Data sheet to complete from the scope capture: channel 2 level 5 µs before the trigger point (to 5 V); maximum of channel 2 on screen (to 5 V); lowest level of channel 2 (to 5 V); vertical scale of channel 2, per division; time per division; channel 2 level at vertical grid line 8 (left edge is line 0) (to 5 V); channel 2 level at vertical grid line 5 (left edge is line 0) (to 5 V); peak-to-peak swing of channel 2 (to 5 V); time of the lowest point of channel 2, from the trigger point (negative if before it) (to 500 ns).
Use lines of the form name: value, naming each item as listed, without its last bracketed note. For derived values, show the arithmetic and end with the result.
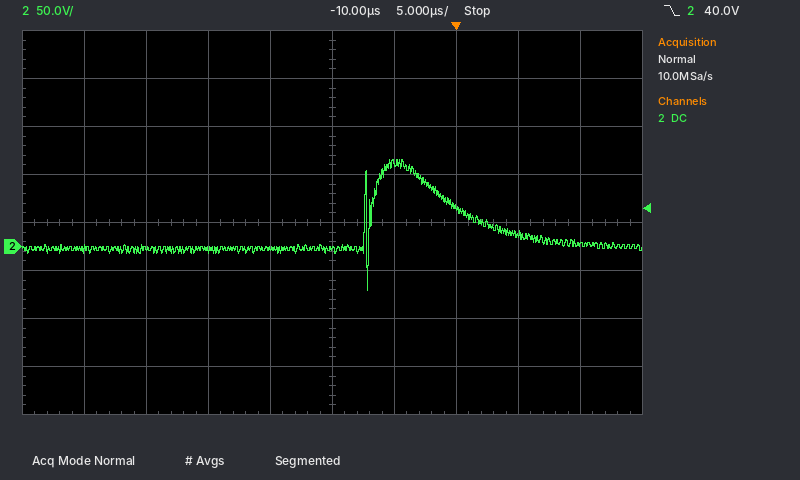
channel 2 level 5 µs before the trigger point: 85 V
maximum of channel 2 on screen: 90 V
lowest level of channel 2: -45 V
vertical scale of channel 2, per division: 50 V
time per division: 5 µs
channel 2 level at vertical grid line 8 (left edge is line 0): 10 V
channel 2 level at vertical grid line 5 (left edge is line 0): -5 V
peak-to-peak swing of channel 2: 90 V − (-45 V) = 135 V
time of the lowest point of channel 2, from the trigger point (negative if before it): -7.0 µs
